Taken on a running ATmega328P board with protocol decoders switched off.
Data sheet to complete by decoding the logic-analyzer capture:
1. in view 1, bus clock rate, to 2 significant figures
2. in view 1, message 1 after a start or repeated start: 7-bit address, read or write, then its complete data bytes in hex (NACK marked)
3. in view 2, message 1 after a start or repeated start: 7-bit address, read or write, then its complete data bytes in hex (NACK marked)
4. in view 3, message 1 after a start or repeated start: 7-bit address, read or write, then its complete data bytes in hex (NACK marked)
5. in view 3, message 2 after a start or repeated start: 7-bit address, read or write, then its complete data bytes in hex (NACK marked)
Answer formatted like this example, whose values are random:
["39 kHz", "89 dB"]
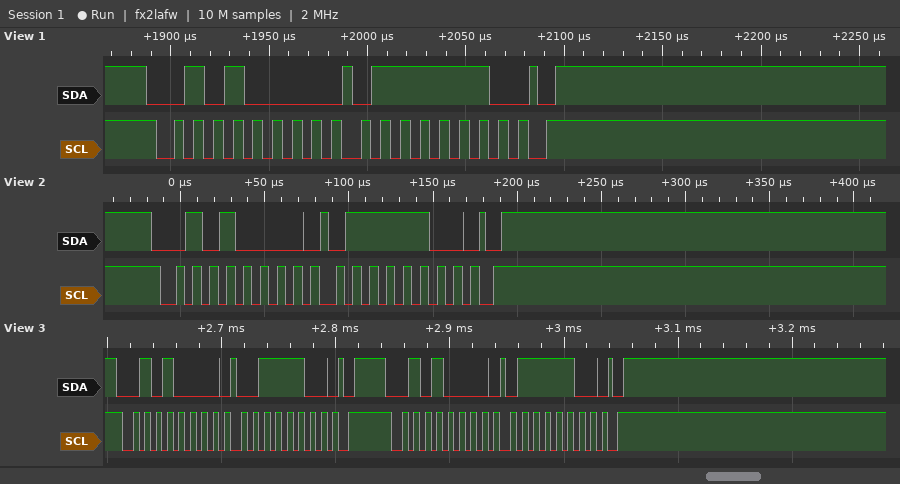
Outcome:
["100 kHz", "0x28 write: 7E", "0x28 write: 7C", "0x28 write: 3C", "0x28 write: 7C"]
